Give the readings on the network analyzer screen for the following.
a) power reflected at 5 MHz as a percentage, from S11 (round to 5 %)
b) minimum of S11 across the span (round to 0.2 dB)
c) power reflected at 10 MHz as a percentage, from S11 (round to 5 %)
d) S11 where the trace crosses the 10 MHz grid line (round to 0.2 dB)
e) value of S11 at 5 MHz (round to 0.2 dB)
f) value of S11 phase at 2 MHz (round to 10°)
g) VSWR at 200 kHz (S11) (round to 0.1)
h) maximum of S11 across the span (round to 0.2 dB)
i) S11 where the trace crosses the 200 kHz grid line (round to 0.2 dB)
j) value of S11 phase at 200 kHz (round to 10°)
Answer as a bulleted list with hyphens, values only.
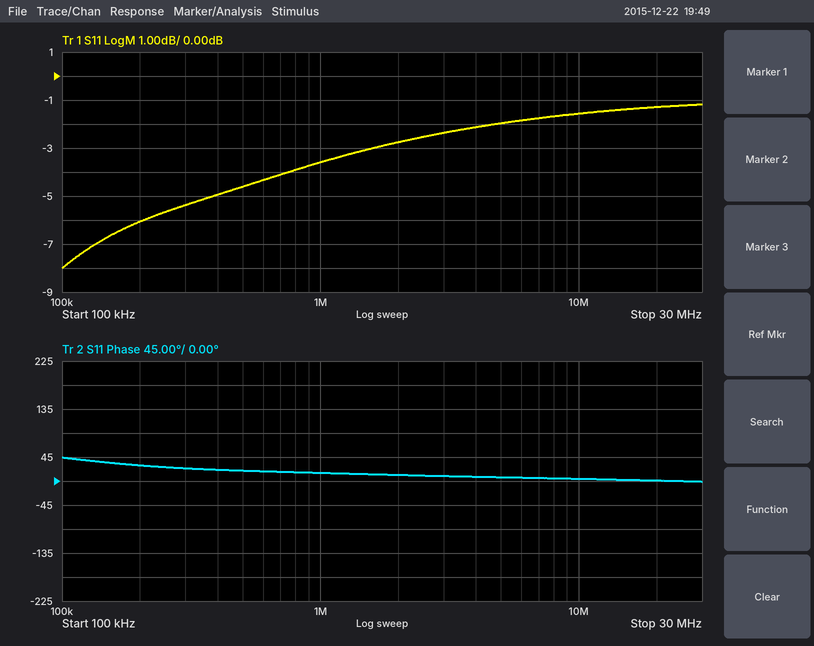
- 65 %
- -8.0 dB
- 70 %
- -1.6 dB
- -2.0 dB
- 10°
- 3.0
- -1.2 dB
- -6.0 dB
- 30°
